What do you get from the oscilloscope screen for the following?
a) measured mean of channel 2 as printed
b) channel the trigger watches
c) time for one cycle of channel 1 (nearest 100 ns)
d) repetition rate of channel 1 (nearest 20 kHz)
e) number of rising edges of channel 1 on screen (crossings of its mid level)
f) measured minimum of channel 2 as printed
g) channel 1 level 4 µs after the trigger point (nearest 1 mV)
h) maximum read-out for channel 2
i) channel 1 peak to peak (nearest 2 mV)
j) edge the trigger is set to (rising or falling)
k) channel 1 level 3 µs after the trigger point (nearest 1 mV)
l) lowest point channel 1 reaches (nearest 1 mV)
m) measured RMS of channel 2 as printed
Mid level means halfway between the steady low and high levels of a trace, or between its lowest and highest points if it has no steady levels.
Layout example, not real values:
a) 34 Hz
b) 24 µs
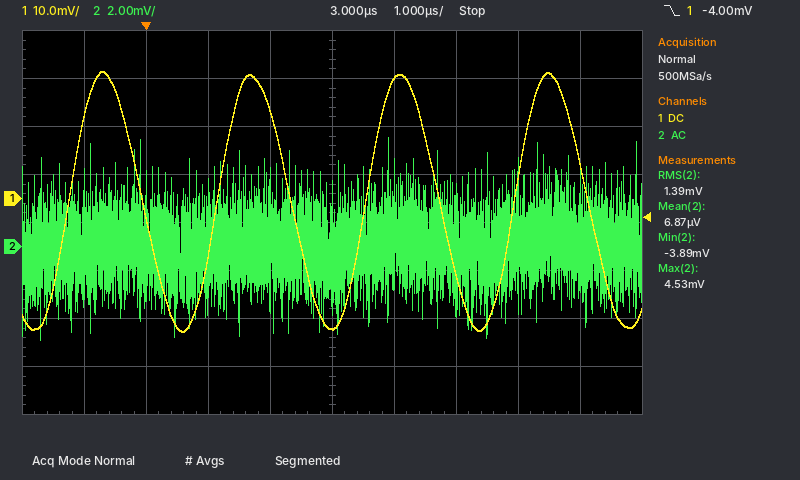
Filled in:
a) 6.87 µV
b) channel 1
c) 2.4 µs
d) 420 kHz
e) 4
f) -3.89 mV
g) 25 mV
h) 4.53 mV
i) 54 mV
j) falling
k) -27 mV
l) -28 mV
m) 1.39 mV
